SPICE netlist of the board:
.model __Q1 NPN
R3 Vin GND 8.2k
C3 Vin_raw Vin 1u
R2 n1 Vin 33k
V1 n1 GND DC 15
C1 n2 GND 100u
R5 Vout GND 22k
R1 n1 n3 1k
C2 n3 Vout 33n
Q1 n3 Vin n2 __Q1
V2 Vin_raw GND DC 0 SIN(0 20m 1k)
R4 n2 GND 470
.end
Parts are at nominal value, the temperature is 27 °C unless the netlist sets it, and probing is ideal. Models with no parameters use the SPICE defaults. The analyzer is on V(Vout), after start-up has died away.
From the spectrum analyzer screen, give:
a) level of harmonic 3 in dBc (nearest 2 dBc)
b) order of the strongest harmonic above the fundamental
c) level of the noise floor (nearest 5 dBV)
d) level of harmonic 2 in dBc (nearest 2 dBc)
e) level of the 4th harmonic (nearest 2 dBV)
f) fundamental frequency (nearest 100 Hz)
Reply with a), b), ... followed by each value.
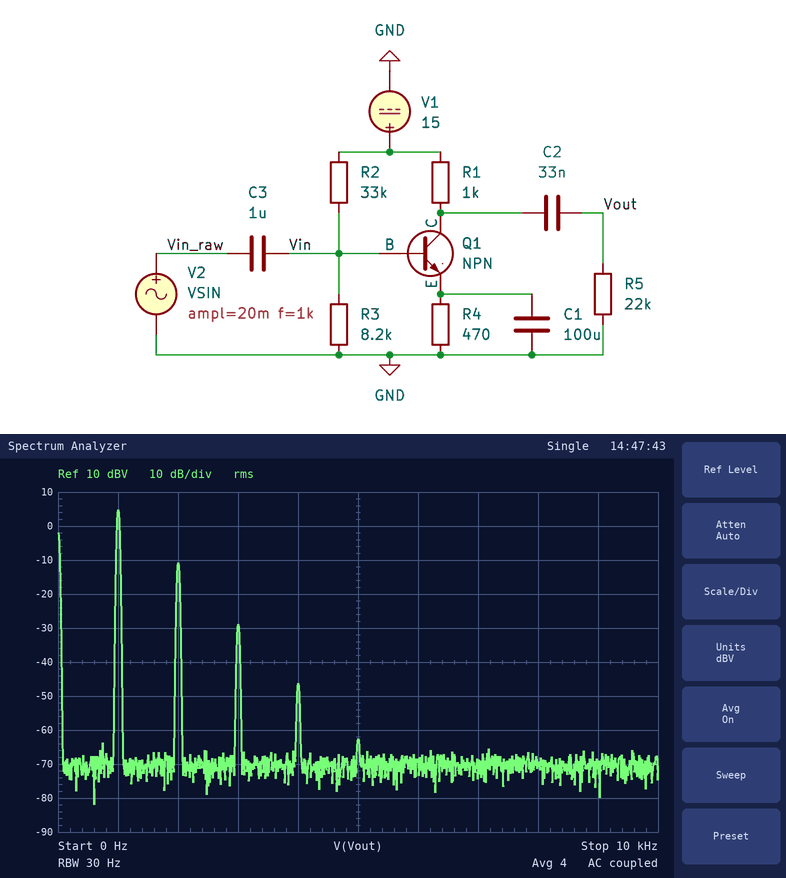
a) -34 dBc
b) 2
c) -70 dBV
d) -16 dBc
e) -46 dBV
f) 1.0 kHz
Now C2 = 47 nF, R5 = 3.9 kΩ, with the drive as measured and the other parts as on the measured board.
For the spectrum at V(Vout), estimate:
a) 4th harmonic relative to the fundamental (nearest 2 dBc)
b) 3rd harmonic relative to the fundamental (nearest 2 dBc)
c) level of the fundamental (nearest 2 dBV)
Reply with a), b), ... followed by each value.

a) -50 dBc
b) -32 dBc
c) 2 dBV
